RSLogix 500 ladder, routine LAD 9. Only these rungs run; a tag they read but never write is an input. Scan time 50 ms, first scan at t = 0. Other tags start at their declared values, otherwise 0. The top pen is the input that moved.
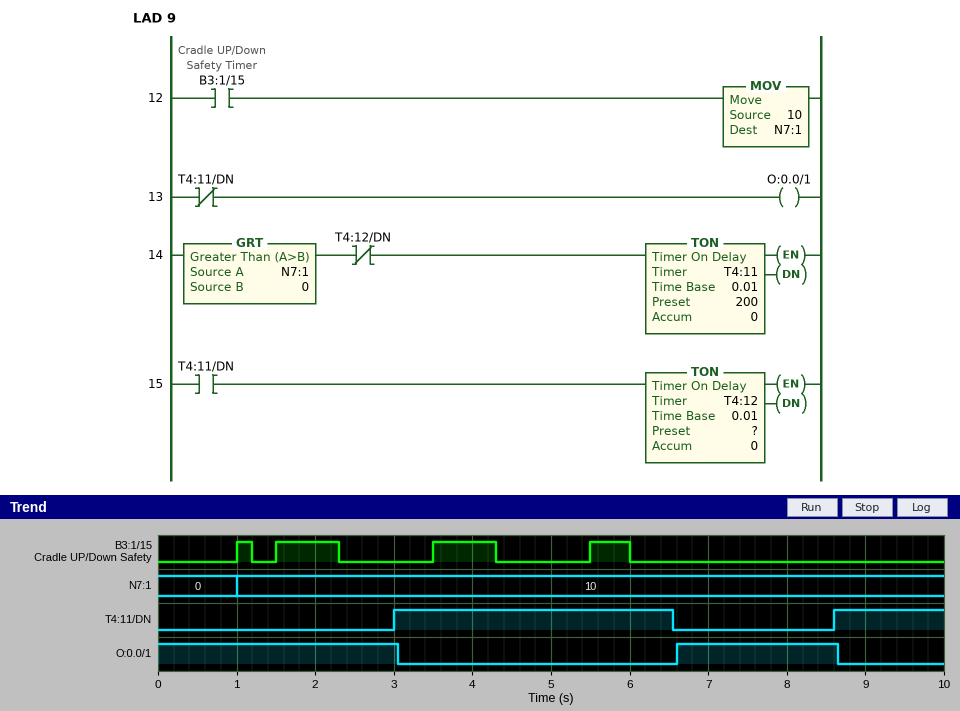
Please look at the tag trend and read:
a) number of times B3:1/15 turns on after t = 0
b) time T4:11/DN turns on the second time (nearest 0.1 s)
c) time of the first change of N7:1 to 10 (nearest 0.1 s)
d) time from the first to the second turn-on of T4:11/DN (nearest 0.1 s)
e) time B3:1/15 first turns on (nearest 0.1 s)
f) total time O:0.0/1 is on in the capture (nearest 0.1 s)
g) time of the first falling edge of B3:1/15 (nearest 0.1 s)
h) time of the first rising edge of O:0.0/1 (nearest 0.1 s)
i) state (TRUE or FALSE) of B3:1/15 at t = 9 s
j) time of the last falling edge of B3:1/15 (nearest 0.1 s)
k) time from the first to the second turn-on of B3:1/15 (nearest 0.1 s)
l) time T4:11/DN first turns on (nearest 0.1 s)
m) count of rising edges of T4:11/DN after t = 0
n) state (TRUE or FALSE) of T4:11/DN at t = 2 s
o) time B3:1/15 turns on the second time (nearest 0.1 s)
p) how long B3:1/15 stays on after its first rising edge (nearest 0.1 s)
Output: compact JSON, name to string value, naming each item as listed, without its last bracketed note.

{"number of times B3:1/15 turns on after t = 0": "4", "time T4:11/DN turns on the second time": "8.6 s", "time of the first change of N7:1 to 10": "1.0 s", "time from the first to the second turn-on of T4:11/DN": "5.6 s", "time B3:1/15 first turns on": "1.0 s", "total time O:0.0/1 is on in the capture": "5.1 s", "time of the first falling edge of B3:1/15": "1.2 s", "time of the first rising edge of O:0.0/1": "6.6 s", "state (TRUE or FALSE) of B3:1/15 at t = 9 s": "FALSE", "time of the last falling edge of B3:1/15": "6.0 s", "time from the first to the second turn-on of B3:1/15": "0.5 s", "time T4:11/DN first turns on": "3.0 s", "count of rising edges of T4:11/DN after t = 0": "2", "state (TRUE or FALSE) of T4:11/DN at t = 2 s": "FALSE", "time B3:1/15 turns on the second time": "1.5 s", "how long B3:1/15 stays on after its first rising edge": "0.2 s"}
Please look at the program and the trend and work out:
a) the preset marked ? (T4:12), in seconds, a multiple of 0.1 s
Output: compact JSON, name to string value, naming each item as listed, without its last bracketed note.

{"the preset marked ? (T4:12), in seconds, a multiple of 0.1 s": "3.5 s"}
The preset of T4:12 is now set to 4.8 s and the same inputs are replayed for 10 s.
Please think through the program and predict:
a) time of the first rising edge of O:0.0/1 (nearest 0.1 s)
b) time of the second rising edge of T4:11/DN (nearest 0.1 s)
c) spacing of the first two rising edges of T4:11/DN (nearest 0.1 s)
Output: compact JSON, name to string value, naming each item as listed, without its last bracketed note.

{"time of the first rising edge of O:0.0/1": "7.9 s", "time of the second rising edge of T4:11/DN": "9.9 s", "spacing of the first two rising edges of T4:11/DN": "6.9 s"}
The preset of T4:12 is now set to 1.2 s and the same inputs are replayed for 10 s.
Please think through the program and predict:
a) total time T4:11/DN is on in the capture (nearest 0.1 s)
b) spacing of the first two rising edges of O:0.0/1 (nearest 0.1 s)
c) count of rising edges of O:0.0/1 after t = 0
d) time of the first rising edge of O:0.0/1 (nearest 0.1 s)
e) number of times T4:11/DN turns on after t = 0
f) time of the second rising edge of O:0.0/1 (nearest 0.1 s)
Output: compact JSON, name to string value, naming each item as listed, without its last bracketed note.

{"total time T4:11/DN is on in the capture": "2.9 s", "spacing of the first two rising edges of O:0.0/1": "3.3 s", "count of rising edges of O:0.0/1 after t = 0": "2", "time of the first rising edge of O:0.0/1": "4.3 s", "number of times T4:11/DN turns on after t = 0": "3", "time of the second rising edge of O:0.0/1": "7.6 s"}
